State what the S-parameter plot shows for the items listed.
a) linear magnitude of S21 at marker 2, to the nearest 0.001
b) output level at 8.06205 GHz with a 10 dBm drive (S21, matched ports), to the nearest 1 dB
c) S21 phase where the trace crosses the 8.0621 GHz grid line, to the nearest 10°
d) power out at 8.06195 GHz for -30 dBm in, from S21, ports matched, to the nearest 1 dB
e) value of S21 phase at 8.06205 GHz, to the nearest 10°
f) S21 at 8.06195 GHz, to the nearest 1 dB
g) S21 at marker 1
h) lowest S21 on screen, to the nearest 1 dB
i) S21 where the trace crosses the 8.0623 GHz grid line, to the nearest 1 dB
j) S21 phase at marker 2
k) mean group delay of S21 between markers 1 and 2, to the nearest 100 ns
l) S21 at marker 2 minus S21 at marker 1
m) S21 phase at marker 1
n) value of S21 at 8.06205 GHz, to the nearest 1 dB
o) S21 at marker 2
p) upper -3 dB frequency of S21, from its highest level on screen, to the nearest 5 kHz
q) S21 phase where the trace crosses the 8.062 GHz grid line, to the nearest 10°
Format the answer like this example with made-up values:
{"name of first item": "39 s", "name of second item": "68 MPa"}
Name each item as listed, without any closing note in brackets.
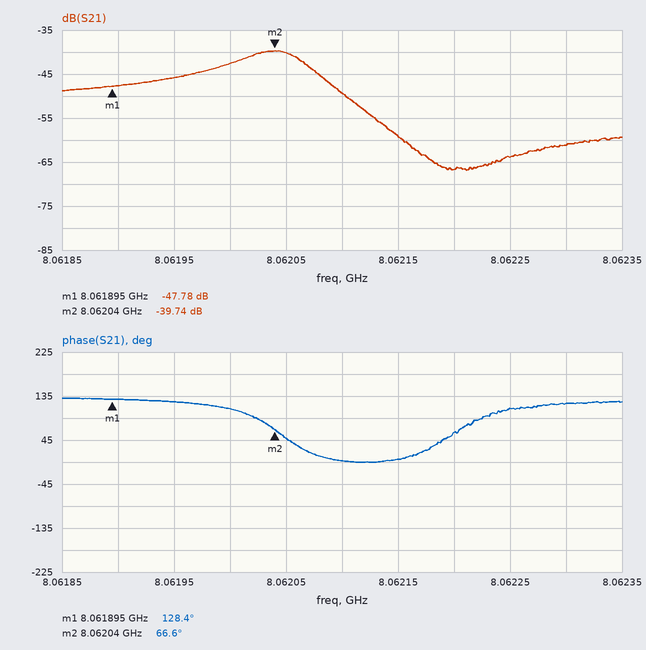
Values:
{"linear magnitude of S21 at marker 2, to the nearest 0.001": "0.010", "output level at 8.06205 GHz with a 10 dBm drive (S21, matched ports), to the nearest 1 dB": "-30 dBm", "S21 phase where the trace crosses the 8.0621 GHz grid line, to the nearest 10°": "0°", "power out at 8.06195 GHz for -30 dBm in, from S21, ports matched, to the nearest 1 dB": "-76 dBm", "value of S21 phase at 8.06205 GHz, to the nearest 10°": "50°", "S21 at 8.06195 GHz, to the nearest 1 dB": "-46 dB", "S21 at marker 1": "-47.78 dB", "lowest S21 on screen, to the nearest 1 dB": "-67 dB", "S21 where the trace crosses the 8.0623 GHz grid line, to the nearest 1 dB": "-61 dB", "S21 phase at marker 2": "66.6°", "mean group delay of S21 between markers 1 and 2, to the nearest 100 ns": "1.2 µs", "S21 at marker 2 minus S21 at marker 1": "8.04 dB", "S21 phase at marker 1": "128.4°", "value of S21 at 8.06205 GHz, to the nearest 1 dB": "-40 dB", "S21 at marker 2": "-39.74 dB", "upper -3 dB frequency of S21, from its highest level on screen, to the nearest 5 kHz": "8.062065 GHz", "S21 phase where the trace crosses the 8.062 GHz grid line, to the nearest 10°": "110°"}
